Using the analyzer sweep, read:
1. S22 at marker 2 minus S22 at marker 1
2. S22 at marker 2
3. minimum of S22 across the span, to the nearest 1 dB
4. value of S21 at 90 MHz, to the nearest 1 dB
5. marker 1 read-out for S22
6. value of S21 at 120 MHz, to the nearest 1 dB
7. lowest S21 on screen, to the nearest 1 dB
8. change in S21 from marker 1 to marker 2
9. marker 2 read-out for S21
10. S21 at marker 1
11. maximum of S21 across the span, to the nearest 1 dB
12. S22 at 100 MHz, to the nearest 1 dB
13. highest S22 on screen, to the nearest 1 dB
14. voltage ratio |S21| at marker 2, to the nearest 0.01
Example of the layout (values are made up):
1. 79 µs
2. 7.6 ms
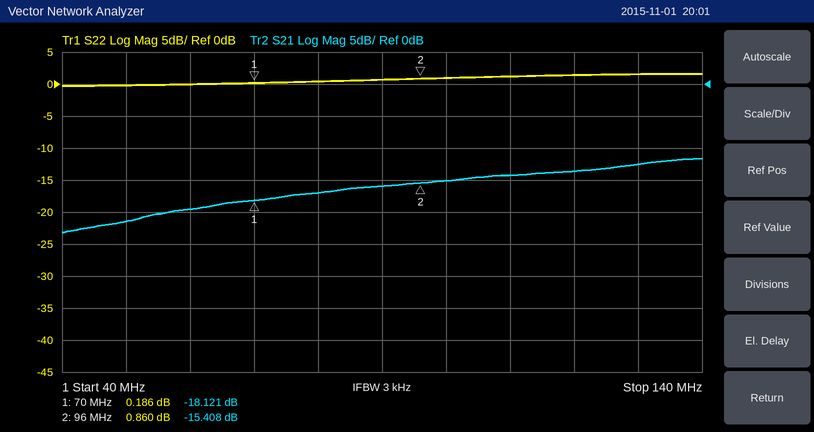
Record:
1. 0.674 dB
2. 0.860 dB
3. 0 dB
4. -16 dB
5. 0.186 dB
6. -14 dB
7. -23 dB
8. 2.713 dB
9. -15.408 dB
10. -18.121 dB
11. -12 dB
12. 1 dB
13. 2 dB
14. 0.17
